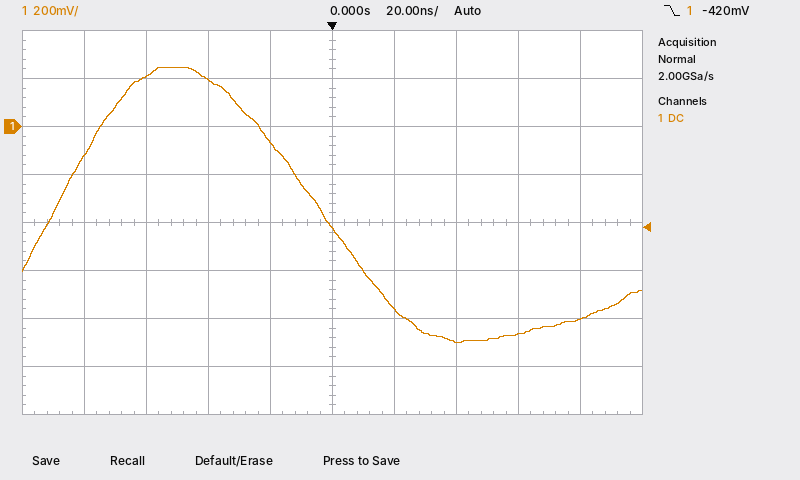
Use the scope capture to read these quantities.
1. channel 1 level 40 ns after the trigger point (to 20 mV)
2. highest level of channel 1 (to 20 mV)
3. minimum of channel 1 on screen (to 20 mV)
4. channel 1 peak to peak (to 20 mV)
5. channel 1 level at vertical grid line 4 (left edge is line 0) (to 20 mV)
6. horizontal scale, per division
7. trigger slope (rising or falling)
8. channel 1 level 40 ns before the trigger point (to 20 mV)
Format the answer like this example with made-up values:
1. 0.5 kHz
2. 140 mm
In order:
1. -900 mV
2. 240 mV
3. -900 mV
4. 1.14 V
5. -60 mV
6. 20 ns
7. falling
8. 200 mV
